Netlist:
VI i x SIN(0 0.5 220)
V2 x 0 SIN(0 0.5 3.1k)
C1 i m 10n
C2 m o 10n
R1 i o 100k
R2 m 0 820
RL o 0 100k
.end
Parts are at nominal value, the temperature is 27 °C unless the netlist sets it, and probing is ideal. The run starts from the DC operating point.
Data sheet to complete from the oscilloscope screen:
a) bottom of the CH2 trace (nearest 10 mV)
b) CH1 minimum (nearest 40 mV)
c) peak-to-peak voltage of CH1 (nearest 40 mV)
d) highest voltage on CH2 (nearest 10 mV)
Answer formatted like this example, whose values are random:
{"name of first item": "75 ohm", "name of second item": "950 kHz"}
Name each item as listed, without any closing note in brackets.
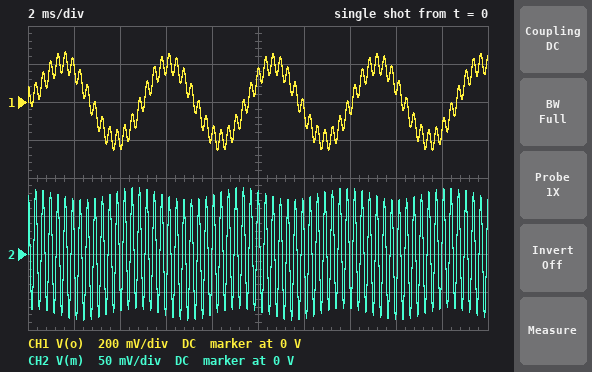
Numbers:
{"bottom of the CH2 trace": "-90 mV", "CH1 minimum": "-240 mV", "peak-to-peak voltage of CH1": "520 mV", "highest voltage on CH2": "90 mV"}
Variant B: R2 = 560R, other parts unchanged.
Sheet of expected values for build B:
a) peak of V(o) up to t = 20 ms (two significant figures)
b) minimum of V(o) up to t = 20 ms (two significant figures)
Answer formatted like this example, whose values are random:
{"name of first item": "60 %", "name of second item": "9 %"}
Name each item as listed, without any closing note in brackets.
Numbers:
{"peak of V(o) up to t = 20 ms": "240 mV", "minimum of V(o) up to t = 20 ms": "-230 mV"}
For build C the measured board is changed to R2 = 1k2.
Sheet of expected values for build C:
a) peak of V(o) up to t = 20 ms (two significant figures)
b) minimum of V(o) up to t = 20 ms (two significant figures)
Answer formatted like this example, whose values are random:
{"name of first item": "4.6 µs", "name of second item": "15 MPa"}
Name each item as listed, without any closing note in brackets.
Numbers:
{"peak of V(o) up to t = 20 ms": "290 mV", "minimum of V(o) up to t = 20 ms": "-280 mV"}
